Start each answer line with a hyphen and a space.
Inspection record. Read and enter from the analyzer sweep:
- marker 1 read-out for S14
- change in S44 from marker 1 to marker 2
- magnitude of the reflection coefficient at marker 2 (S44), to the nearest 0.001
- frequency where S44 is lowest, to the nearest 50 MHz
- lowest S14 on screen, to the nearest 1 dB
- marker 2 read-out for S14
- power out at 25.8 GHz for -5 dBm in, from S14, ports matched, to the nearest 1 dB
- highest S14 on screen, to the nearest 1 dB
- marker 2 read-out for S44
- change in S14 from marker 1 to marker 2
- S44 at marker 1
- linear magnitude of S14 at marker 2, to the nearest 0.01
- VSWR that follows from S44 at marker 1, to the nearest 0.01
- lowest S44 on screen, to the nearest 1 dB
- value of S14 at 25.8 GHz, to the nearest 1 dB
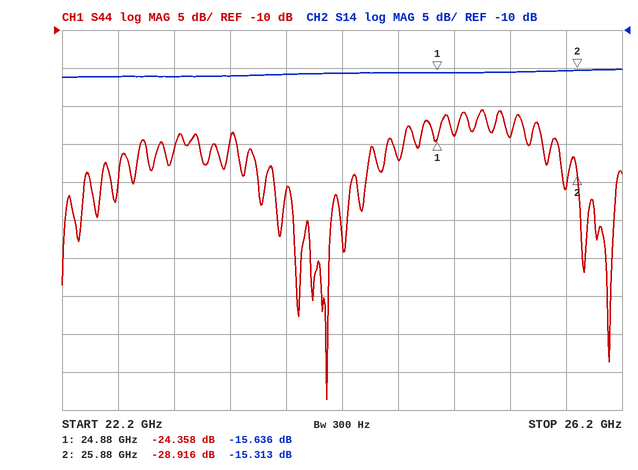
- -15.636 dB
- -4.558 dB
- 0.036
- 24.10 GHz
- -16 dB
- -15.313 dB
- -20 dBm
- -15 dB
- -28.916 dB
- 0.323 dB
- -24.358 dB
- 0.17
- 1.13
- -59 dB
- -15 dB
